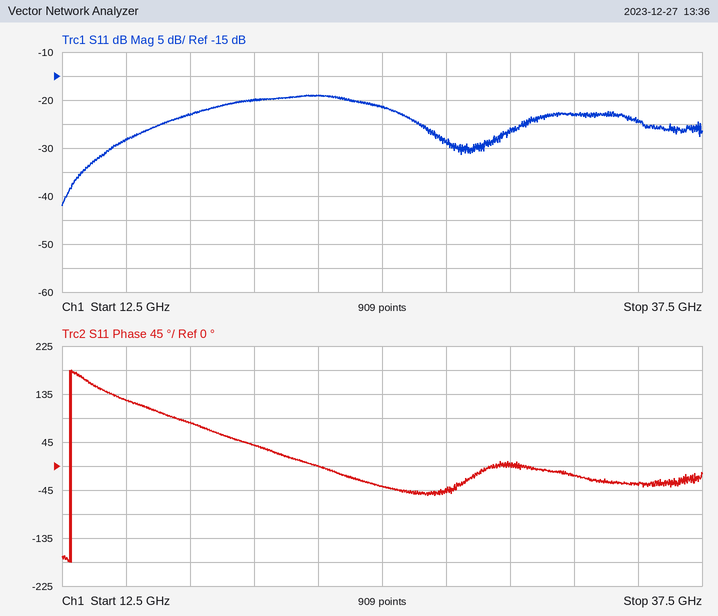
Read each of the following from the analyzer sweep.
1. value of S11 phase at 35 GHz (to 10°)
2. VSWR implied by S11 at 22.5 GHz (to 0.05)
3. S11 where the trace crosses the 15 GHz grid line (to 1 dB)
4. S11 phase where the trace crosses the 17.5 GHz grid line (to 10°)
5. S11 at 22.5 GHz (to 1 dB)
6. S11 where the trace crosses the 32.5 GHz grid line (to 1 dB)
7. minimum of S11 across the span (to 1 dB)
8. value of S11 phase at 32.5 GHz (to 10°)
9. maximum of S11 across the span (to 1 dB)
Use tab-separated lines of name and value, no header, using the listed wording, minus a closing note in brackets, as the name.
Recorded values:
value of S11 phase at 35 GHz	-30°
VSWR implied by S11 at 22.5 GHz	1.25
S11 where the trace crosses the 15 GHz grid line	-28 dB
S11 phase where the trace crosses the 17.5 GHz grid line	80°
S11 at 22.5 GHz	-19 dB
S11 where the trace crosses the 32.5 GHz grid line	-23 dB
minimum of S11 across the span	-42 dB
value of S11 phase at 32.5 GHz	-20°
maximum of S11 across the span	-19 dB
